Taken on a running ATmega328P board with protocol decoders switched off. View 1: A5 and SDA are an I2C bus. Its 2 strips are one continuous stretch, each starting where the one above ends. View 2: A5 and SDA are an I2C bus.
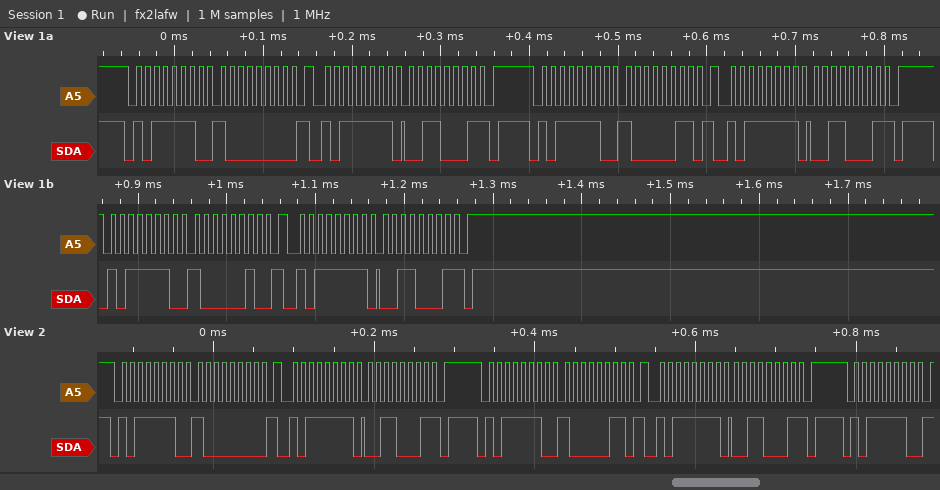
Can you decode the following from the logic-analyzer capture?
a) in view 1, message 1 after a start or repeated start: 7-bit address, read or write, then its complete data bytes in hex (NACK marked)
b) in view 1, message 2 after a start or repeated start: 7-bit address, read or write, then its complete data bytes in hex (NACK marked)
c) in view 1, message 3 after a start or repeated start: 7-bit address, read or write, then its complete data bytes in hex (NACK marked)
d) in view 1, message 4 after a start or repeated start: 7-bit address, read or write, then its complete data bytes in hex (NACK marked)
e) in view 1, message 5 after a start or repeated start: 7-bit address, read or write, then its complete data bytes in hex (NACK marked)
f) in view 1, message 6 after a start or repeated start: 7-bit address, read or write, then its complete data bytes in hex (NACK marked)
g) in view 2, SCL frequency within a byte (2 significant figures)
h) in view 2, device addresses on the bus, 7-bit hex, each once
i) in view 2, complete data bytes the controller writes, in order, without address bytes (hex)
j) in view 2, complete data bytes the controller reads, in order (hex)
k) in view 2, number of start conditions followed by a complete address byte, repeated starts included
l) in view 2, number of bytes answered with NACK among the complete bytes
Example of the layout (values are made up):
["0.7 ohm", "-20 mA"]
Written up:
["0x5F write: 80", "0x5F read: 31 NACK", "0x5F write: 83", "0x5F read: 31 NACK", "0x5F write: 82", "0x5F read: 31 NACK", "100 kHz", "0x5F", "80 83", "31 31", "5", "2"]
